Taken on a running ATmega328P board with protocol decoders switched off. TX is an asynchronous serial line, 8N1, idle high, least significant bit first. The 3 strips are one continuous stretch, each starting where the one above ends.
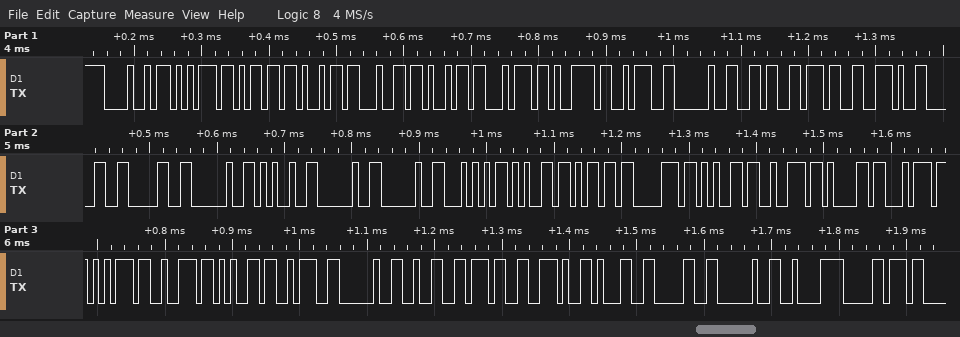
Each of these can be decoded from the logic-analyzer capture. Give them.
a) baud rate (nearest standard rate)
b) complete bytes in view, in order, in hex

115200 baud
0x48 0x75 0x6D 0x69 0x64 0x69 0x74 0x79 0x3A 0x20 0x36 0x37 0x2E 0x30 0x30 0x20 0x25 0x20 0x20 0x54 0x65 0x6D 0x70 0x65 0x72 0x61 0x74 0x75 0x72 0x65 0x3A 0x20 0x32 0x37 0x2E 0x31 0x30 0x20 0xC2 0xB0
